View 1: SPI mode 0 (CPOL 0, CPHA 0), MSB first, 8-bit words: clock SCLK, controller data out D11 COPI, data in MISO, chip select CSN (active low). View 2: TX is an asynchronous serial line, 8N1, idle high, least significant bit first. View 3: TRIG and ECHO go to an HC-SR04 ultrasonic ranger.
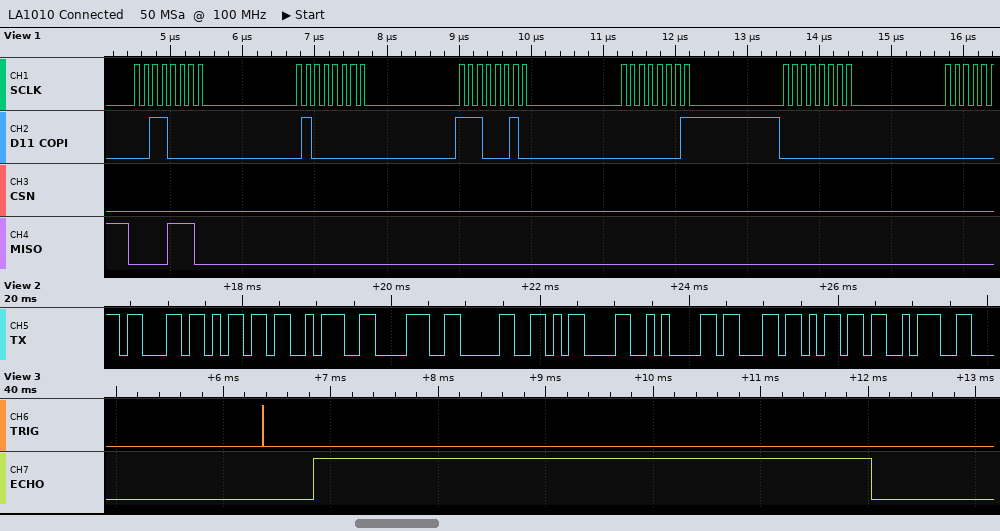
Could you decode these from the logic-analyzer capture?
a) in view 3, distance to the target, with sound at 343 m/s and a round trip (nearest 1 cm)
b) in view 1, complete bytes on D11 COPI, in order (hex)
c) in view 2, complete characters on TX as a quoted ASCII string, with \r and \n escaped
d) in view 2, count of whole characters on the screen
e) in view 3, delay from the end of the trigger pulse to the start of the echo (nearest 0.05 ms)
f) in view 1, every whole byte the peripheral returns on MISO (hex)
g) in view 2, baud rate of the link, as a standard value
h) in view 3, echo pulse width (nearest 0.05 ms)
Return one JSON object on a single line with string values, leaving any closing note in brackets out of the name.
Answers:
{"in view 3, distance to the target, with sound at 343 m/s and a round trip": "89 cm", "in view 1, complete bytes on D11 COPI, in order": "30 40 E2 01 00", "in view 2, complete characters on TX as a quoted ASCII string, with \\r and \\n escaped": "\"cm:80\\r\\ncm:\"", "in view 2, count of whole characters on the screen": "10", "in view 3, delay from the end of the trigger pulse to the start of the echo": "0.45 ms", "in view 1, every whole byte the peripheral returns on MISO": "0E 00 00 00 00", "in view 2, baud rate of the link, as a standard value": "9600 baud", "in view 3, echo pulse width": "5.20 ms"}
